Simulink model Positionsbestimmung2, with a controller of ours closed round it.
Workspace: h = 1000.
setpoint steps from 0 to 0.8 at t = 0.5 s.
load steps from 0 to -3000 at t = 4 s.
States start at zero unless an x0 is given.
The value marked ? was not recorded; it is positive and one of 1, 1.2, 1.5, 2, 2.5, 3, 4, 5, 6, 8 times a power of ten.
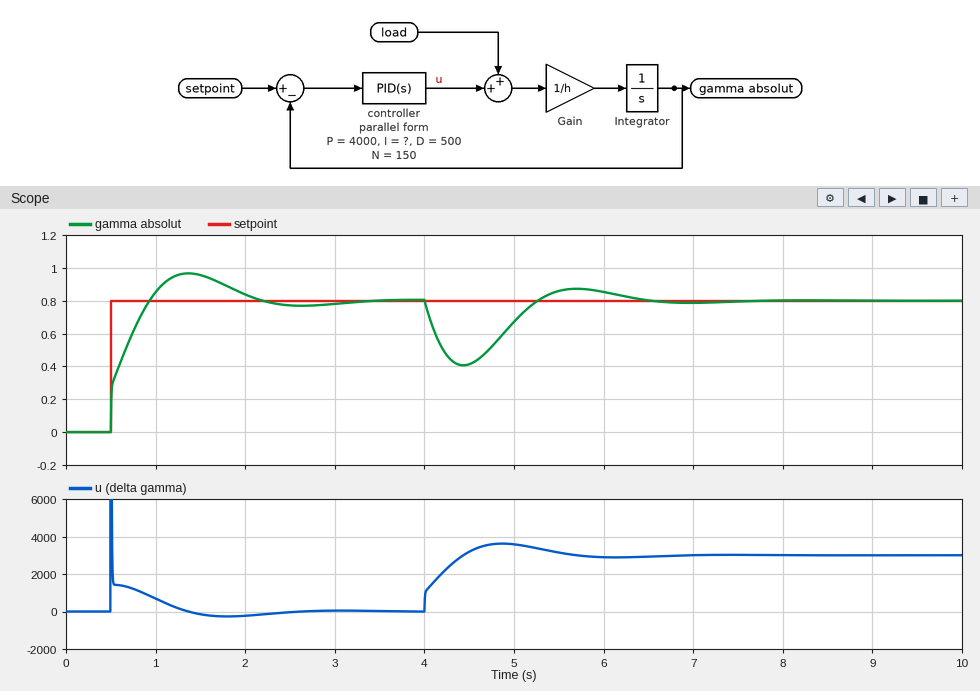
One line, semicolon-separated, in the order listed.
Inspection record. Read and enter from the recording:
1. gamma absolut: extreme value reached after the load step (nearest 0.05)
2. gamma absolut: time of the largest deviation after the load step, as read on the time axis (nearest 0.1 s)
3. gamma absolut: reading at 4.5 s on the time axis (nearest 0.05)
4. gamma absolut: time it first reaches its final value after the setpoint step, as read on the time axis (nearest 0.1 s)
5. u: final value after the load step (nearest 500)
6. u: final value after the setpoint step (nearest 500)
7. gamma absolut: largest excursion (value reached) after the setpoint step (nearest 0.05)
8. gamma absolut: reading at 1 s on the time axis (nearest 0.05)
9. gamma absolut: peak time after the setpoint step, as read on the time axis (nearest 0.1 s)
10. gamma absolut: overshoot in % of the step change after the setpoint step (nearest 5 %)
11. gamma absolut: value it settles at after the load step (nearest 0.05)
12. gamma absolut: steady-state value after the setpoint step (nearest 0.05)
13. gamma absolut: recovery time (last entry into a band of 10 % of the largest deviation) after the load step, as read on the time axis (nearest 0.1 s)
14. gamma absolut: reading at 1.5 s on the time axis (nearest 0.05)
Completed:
0.40; 4.4 s; 0.40; 0.9 s; 3000; 0; 0.95; 0.85; 1.4 s; 20 %; 0.80; 0.80; 6.1 s; 0.95
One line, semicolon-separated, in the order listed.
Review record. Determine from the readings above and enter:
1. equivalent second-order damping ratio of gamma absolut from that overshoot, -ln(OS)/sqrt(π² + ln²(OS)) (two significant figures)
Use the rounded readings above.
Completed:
0.46
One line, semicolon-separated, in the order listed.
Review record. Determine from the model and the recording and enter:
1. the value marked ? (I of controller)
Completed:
12000
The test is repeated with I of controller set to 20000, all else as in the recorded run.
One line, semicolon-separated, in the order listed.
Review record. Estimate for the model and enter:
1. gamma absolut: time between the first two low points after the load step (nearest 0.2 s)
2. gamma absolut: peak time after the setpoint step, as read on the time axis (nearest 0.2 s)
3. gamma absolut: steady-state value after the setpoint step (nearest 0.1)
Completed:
1.8 s; 1.2 s; 0.8
